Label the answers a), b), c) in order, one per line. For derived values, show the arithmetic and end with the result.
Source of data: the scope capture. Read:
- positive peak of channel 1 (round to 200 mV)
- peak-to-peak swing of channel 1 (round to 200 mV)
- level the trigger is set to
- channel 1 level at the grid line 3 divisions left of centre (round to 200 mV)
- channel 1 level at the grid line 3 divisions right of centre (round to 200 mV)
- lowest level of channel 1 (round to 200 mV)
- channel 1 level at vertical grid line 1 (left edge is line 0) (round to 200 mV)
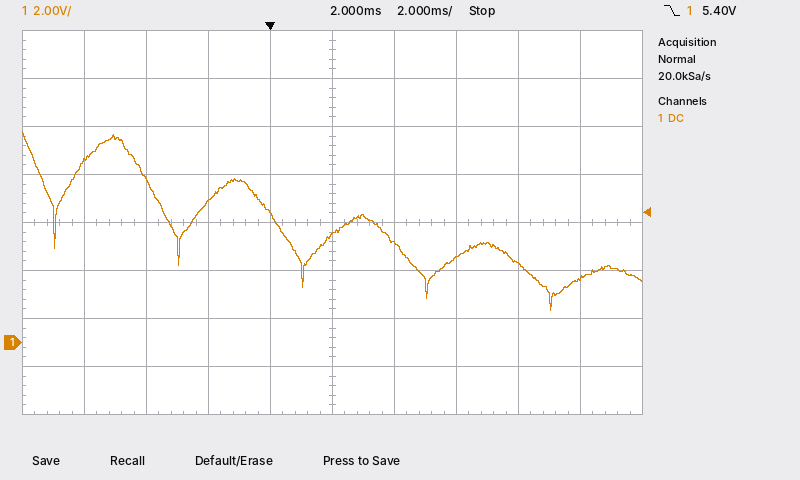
a) 8.8 V
b) 8.8 V − (1.4 V) = 7.4 V
c) 5.40 V
d) 6.8 V
e) 3.2 V
f) 1.4 V
g) 7.6 V
